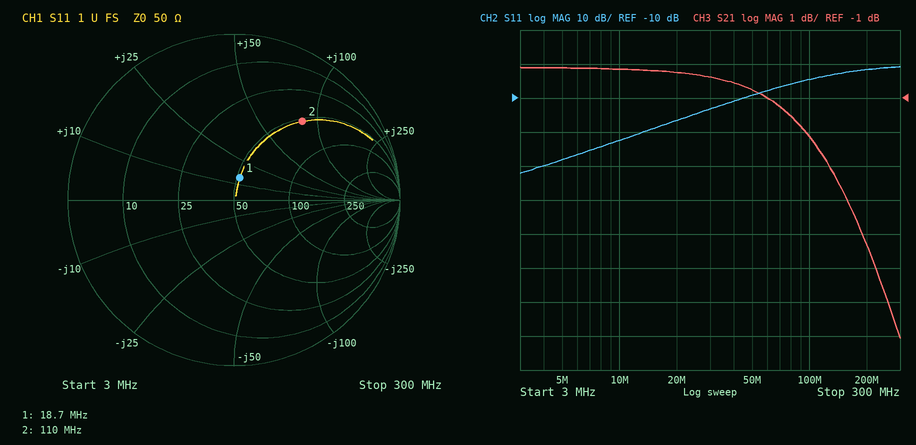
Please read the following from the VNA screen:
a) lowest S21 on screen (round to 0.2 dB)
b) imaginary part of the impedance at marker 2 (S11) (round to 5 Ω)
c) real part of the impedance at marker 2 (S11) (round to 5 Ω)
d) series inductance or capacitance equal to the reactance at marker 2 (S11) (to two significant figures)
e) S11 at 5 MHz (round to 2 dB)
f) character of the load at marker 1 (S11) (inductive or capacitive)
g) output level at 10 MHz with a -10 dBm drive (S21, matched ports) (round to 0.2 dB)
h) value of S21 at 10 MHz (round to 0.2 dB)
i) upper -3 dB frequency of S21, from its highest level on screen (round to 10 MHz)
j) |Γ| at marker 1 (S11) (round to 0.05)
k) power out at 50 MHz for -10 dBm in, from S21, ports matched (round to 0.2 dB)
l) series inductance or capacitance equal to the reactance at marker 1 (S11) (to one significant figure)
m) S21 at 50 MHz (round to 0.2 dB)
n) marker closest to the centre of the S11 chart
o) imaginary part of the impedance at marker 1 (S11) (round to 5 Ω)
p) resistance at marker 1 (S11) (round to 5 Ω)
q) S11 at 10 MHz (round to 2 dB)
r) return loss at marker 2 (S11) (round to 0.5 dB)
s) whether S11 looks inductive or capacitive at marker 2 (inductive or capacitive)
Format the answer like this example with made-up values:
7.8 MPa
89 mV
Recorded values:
-8.0 dB
+85 Ω
55 Ω
120 nH
-28 dB
inductive
-10.2 dBm
-0.2 dB
130 MHz
0.15
-10.8 dBm
100 nH
-0.8 dB
marker 1
+15 Ω
50 Ω
-22 dB
4.0 dB
inductive
